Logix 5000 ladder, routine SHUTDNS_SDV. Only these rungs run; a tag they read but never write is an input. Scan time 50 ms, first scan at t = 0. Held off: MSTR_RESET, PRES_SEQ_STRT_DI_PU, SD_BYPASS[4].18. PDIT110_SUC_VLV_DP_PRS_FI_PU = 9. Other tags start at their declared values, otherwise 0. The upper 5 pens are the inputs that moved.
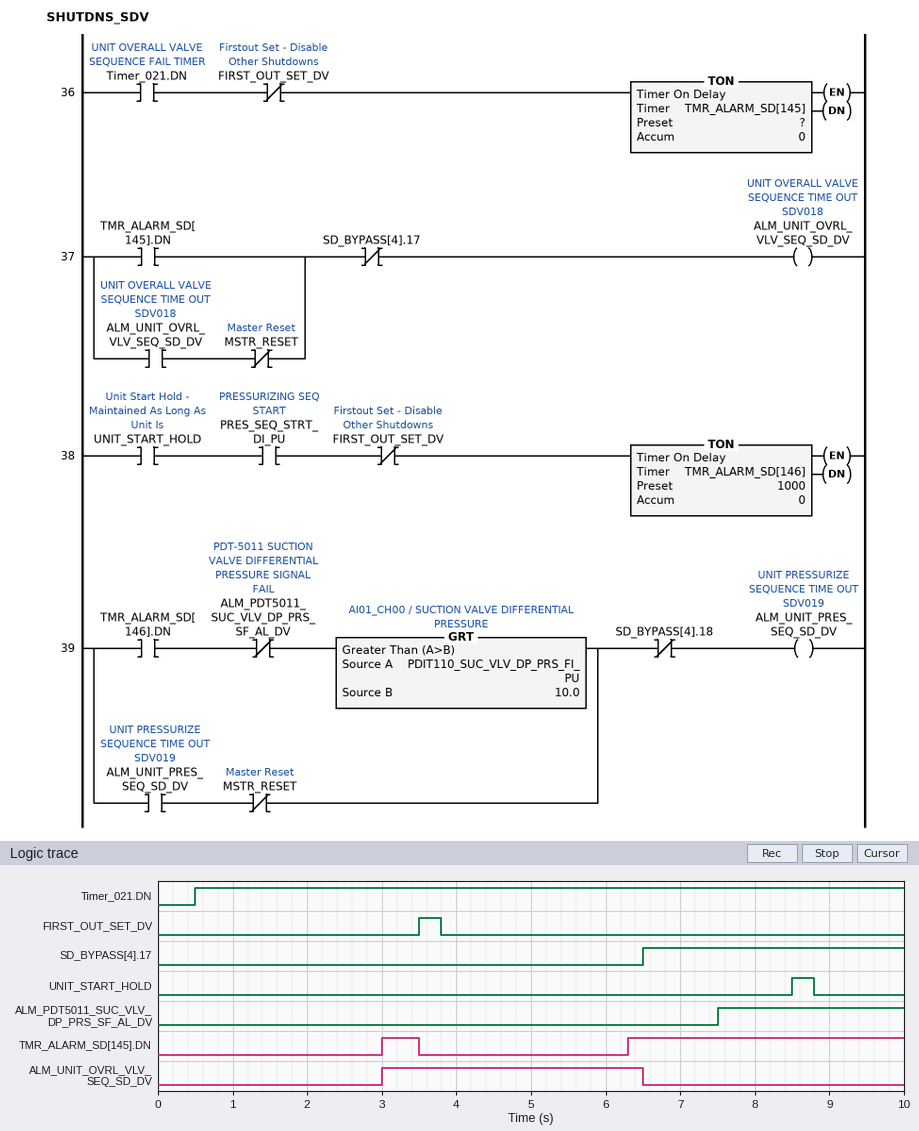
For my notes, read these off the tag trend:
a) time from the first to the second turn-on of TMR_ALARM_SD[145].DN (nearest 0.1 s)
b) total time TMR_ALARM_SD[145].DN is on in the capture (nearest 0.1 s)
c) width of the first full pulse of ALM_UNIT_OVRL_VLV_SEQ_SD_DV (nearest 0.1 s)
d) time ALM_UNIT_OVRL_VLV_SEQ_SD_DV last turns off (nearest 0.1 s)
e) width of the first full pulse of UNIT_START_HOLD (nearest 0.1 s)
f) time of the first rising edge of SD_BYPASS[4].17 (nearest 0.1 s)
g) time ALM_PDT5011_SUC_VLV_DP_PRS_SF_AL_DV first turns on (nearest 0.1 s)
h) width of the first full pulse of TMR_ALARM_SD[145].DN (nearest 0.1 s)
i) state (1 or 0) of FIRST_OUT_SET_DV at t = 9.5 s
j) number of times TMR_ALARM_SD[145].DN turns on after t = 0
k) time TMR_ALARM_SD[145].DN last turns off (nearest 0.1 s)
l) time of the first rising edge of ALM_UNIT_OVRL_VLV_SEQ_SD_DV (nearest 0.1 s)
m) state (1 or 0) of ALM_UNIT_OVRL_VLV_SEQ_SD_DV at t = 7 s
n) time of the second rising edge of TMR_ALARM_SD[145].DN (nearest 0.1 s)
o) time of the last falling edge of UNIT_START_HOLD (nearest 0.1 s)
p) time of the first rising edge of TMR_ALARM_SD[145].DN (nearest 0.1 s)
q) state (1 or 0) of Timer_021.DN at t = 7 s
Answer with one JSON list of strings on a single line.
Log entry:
["3.3 s", "4.2 s", "3.5 s", "6.5 s", "0.3 s", "6.5 s", "7.5 s", "0.5 s", "0", "2", "3.5 s", "3.0 s", "0", "6.3 s", "8.8 s", "3.0 s", "1"]
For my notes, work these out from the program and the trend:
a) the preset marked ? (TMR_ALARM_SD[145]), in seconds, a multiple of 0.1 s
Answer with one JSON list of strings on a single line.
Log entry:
["2.5 s"]
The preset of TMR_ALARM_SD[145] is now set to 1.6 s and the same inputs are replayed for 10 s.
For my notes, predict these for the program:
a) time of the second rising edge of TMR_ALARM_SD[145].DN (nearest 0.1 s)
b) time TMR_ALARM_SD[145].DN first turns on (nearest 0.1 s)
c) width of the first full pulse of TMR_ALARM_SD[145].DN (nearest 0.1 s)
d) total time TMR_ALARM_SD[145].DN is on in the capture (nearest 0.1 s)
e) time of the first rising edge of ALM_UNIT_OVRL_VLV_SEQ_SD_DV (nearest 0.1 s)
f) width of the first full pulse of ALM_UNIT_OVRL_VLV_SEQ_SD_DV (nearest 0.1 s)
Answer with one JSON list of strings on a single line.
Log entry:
["5.4 s", "2.1 s", "1.4 s", "6.0 s", "2.1 s", "4.4 s"]
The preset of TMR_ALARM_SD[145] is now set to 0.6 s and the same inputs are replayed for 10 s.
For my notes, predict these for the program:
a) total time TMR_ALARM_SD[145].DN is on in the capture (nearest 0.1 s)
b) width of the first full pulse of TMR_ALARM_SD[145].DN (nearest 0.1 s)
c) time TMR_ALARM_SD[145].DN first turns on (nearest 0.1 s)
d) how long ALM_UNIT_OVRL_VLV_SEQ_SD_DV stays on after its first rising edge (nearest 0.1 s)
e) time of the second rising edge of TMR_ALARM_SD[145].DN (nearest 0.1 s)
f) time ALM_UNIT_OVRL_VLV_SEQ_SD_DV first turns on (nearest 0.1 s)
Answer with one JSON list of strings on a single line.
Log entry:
["8.0 s", "2.4 s", "1.1 s", "5.4 s", "4.4 s", "1.1 s"]
